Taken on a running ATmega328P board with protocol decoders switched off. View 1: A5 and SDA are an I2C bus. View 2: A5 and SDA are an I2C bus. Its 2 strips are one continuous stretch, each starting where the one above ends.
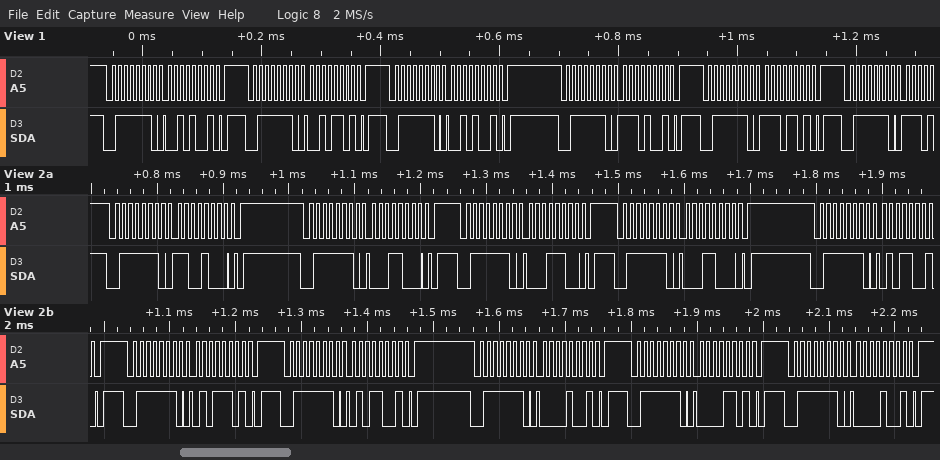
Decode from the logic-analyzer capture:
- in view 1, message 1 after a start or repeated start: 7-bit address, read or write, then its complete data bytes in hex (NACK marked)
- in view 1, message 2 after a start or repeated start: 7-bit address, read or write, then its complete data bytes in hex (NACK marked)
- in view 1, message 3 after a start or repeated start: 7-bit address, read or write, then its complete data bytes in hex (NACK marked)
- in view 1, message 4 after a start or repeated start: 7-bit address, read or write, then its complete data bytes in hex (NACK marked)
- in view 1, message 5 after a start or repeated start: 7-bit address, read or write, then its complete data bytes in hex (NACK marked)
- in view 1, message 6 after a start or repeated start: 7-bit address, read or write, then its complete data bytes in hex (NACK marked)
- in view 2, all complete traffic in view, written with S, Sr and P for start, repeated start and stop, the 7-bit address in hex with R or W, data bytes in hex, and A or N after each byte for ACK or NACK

0x3F write: 29
0x3F write: 2D
0x3F write: 29
0x3F write: E9
0x3F write: ED
0x3F write
S 3FW A C8 A P S 3FW A 18 A P S 3FW A 1C A P S 3FW A 18 A P S 3FW A 59 A P S 3FW A 5D A P S 3FW A 59 A P S 3FW A 09 A P S 3FW A 0D A P S 3FW A 09 A P
